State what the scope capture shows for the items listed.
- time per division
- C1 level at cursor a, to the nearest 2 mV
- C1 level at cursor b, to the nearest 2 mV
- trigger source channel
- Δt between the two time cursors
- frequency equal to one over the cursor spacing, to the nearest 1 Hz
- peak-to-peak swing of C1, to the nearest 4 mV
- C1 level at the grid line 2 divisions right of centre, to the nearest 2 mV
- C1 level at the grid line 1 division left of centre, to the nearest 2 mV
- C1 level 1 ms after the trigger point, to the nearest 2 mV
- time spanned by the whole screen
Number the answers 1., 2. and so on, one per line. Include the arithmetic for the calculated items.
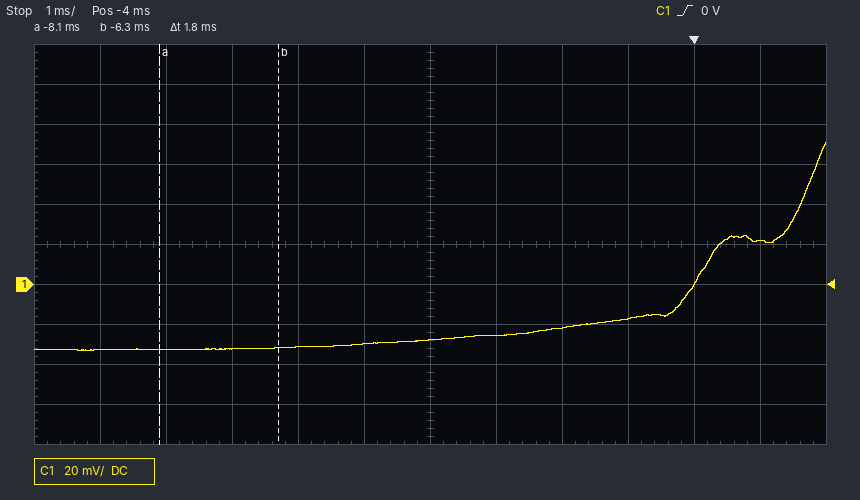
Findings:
1. 1 ms
2. -32 mV
3. -32 mV
4. C1
5. 1.8 ms
6. 1 / 1.8 ms ≈ 556 Hz
7. 104 mV
8. -22 mV
9. -30 mV
10. 22 mV
11. 12 ms
